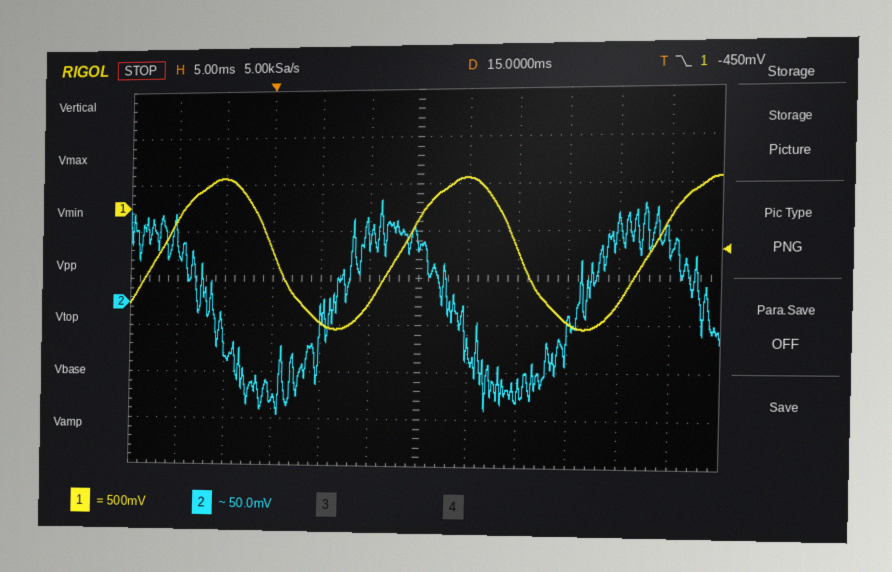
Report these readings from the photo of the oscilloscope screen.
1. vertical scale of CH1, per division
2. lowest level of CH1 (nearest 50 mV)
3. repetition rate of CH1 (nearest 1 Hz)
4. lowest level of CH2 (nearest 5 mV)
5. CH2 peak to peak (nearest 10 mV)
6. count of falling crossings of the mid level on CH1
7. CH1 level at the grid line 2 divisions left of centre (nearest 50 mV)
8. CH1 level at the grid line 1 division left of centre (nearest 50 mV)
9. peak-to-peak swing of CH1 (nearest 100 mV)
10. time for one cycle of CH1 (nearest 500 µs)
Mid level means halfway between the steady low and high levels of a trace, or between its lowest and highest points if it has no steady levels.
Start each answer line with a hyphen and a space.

- 500 mV
- -1.30 V
- 40 Hz
- -120 mV
- 230 mV
- 2
- -1.20 V
- -1.00 V
- 1.60 V
- 25.0 ms
